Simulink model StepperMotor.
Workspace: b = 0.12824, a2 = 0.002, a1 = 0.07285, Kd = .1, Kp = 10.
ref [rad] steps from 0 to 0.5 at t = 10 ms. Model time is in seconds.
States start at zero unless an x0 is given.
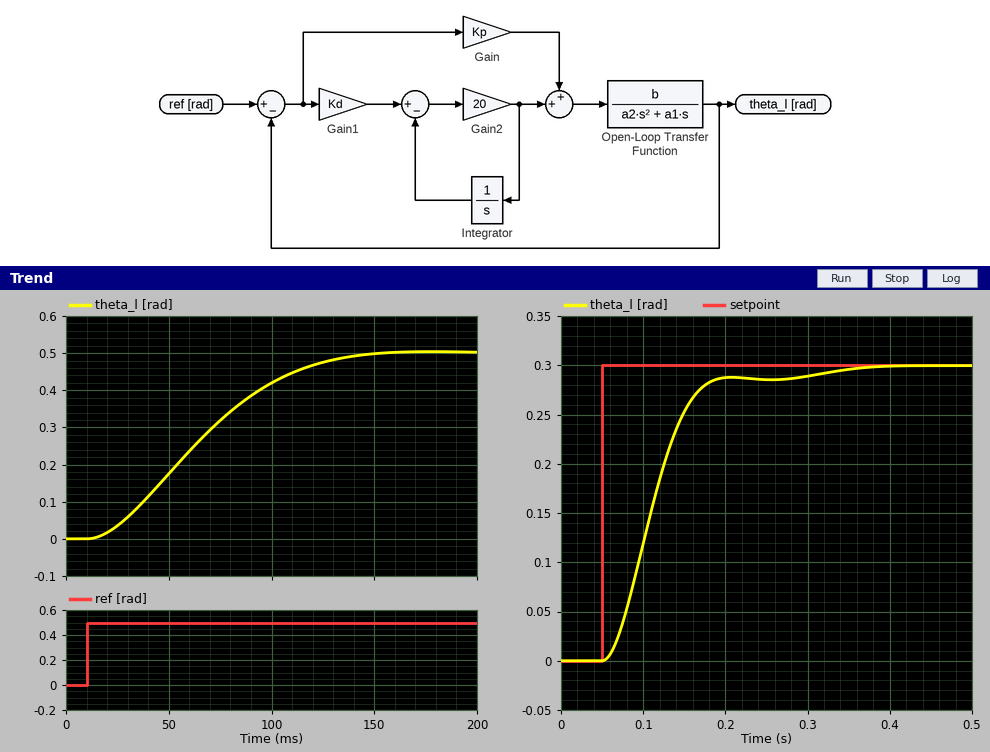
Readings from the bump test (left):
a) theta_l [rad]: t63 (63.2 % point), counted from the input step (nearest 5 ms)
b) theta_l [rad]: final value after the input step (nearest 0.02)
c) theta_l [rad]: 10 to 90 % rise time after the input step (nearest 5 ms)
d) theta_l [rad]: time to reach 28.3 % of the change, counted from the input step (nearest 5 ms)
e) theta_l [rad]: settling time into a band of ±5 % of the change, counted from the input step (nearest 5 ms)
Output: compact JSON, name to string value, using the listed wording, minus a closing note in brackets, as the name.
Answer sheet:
{"theta_l [rad]: t63 (63.2 % point), counted from the input step": "65 ms", "theta_l [rad]: final value after the input step": "0.50", "theta_l [rad]: 10 to 90 % rise time after the input step": "85 ms", "theta_l [rad]: time to reach 28.3 % of the change, counted from the input step": "35 ms", "theta_l [rad]: settling time into a band of ±5 % of the change, counted from the input step": "115 ms"}
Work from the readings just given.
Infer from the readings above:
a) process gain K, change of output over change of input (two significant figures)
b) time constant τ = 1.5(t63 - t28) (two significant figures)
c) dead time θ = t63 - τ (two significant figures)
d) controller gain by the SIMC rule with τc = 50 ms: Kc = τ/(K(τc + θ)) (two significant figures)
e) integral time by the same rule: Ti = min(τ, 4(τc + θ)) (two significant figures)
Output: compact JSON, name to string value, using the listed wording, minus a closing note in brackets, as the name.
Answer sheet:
{"process gain K, change of output over change of input": "1.0", "time constant τ = 1.5(t63 - t28)": "45 ms", "dead time θ = t63 - τ": "20 ms", "controller gain by the SIMC rule with τc = 50 ms: Kc = τ/(K(τc + θ))": "0.64", "integral time by the same rule: Ti = min(τ, 4(τc + θ))": "45 ms"}
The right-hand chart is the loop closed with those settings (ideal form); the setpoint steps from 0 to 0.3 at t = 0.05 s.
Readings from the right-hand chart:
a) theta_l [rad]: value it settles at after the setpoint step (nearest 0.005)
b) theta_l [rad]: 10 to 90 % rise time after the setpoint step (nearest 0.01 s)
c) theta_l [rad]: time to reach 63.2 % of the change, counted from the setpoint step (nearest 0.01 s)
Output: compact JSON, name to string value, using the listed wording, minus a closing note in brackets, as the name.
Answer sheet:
{"theta_l [rad]: value it settles at after the setpoint step": "0.300", "theta_l [rad]: 10 to 90 % rise time after the setpoint step": "0.09 s", "theta_l [rad]: time to reach 63.2 % of the change, counted from the setpoint step": "0.07 s"}
